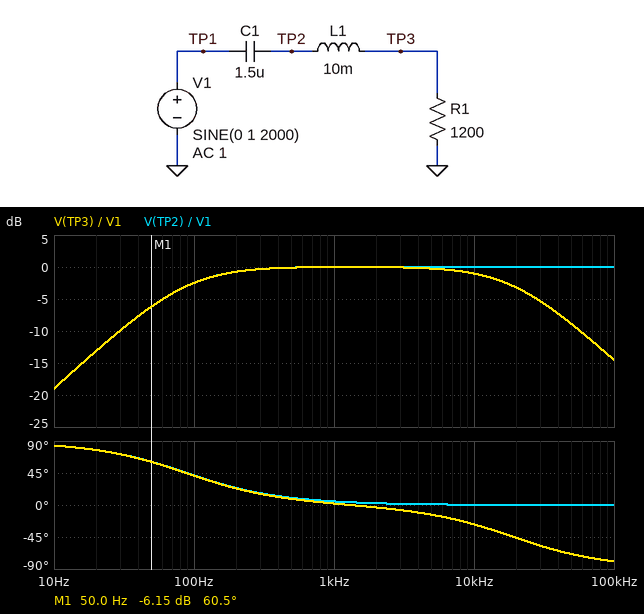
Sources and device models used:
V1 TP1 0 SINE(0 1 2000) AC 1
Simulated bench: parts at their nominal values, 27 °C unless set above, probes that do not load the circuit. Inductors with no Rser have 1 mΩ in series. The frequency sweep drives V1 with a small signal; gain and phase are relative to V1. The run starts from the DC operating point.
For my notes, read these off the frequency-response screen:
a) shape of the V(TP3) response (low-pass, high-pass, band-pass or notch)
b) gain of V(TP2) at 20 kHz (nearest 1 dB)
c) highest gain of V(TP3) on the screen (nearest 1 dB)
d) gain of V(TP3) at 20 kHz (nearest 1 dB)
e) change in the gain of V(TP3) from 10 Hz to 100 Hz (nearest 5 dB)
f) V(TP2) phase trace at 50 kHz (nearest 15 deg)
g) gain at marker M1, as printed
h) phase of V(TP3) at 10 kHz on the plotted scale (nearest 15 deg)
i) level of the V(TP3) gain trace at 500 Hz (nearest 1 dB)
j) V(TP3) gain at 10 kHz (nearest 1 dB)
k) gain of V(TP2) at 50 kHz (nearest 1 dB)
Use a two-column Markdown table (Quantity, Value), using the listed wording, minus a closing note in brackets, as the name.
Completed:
| Quantity | Value |
|---|---|
| shape of the V(TP3) response | band-pass |
| gain of V(TP2) at 20 kHz | 0 dB |
| highest gain of V(TP3) on the screen | 0 dB |
| gain of V(TP3) at 20 kHz | -3 dB |
| change in the gain of V(TP3) from 10 Hz to 100 Hz | 15 dB |
| V(TP2) phase trace at 50 kHz | 0 deg |
| gain at marker M1, as printed | -6.15 dB |
| phase of V(TP3) at 10 kHz on the plotted scale | -30 deg |
| level of the V(TP3) gain trace at 500 Hz | 0 dB |
| V(TP3) gain at 10 kHz | -1 dB |
| gain of V(TP2) at 50 kHz | 0 dB |
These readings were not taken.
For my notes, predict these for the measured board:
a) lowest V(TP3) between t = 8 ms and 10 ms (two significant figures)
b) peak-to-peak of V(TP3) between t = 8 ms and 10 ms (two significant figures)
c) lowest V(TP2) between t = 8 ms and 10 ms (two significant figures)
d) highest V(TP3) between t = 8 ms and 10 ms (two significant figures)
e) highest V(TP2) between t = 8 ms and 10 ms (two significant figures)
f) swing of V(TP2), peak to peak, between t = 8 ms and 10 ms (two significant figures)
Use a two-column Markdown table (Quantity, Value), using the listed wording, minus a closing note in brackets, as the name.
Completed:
| Quantity | Value |
|---|---|
| lowest V(TP3) between t = 8 ms and 10 ms | -1.0 V |
| peak-to-peak of V(TP3) between t = 8 ms and 10 ms | 2.0 V |
| lowest V(TP2) between t = 8 ms and 10 ms | -1.0 V |
| highest V(TP3) between t = 8 ms and 10 ms | 1.0 V |
| highest V(TP2) between t = 8 ms and 10 ms | 1.0 V |
| swing of V(TP2), peak to peak, between t = 8 ms and 10 ms | 2.0 V |
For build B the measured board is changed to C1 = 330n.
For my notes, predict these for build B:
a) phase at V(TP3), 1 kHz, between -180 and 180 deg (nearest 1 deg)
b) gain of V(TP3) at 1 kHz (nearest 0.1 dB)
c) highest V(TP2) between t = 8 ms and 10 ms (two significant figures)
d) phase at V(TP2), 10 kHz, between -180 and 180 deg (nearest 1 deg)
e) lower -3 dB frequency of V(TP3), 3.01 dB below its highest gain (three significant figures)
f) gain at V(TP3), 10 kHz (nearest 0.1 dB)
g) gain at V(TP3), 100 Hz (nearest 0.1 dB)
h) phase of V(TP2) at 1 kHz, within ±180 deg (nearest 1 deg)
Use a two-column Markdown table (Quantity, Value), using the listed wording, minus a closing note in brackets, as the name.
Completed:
| Quantity | Value |
|---|---|
| phase at V(TP3), 1 kHz, between -180 and 180 deg | 19 deg |
| gain of V(TP3) at 1 kHz | -0.5 dB |
| highest V(TP2) between t = 8 ms and 10 ms | 1.0 V |
| phase at V(TP2), 10 kHz, between -180 and 180 deg | 2 deg |
| lower -3 dB frequency of V(TP3), 3.01 dB below its highest gain | 394 Hz |
| gain at V(TP3), 10 kHz | -0.9 dB |
| gain at V(TP3), 100 Hz | -12.3 dB |
| phase of V(TP2) at 1 kHz, within ±180 deg | 22 deg |
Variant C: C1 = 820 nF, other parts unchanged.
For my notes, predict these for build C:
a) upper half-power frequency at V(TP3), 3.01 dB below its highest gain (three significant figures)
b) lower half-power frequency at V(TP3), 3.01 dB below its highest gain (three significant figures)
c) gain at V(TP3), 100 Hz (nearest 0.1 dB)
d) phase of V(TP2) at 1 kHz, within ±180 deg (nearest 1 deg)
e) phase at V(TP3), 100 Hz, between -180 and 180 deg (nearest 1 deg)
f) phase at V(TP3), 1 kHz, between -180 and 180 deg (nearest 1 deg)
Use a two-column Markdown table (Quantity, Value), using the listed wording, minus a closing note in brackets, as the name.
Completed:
| Quantity | Value |
|---|---|
| upper half-power frequency at V(TP3), 3.01 dB below its highest gain | 19.3 kHz |
| lower half-power frequency at V(TP3), 3.01 dB below its highest gain | 160 Hz |
| gain at V(TP3), 100 Hz | -5.6 dB |
| phase of V(TP2) at 1 kHz, within ±180 deg | 9 deg |
| phase at V(TP3), 100 Hz, between -180 and 180 deg | 58 deg |
| phase at V(TP3), 1 kHz, between -180 and 180 deg | 6 deg |
